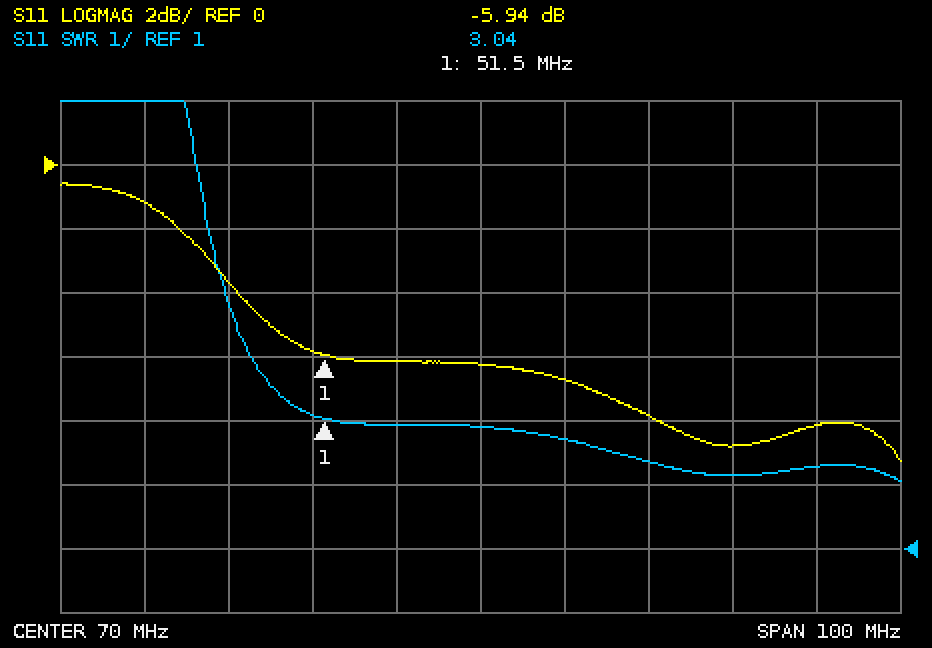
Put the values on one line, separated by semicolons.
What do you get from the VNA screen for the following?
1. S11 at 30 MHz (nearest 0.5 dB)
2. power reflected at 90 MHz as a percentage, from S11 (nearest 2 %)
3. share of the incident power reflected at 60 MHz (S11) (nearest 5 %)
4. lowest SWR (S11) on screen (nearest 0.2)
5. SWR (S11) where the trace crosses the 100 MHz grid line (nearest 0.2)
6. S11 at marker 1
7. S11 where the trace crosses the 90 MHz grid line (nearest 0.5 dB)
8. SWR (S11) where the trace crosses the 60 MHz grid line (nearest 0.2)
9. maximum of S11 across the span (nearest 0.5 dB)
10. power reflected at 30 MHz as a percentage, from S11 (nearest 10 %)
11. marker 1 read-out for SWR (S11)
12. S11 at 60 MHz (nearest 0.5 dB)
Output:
-1.0 dB; 16 %; 25 %; 2.0; 2.2; -5.94 dB; -8.0 dB; 3.0; -0.5 dB; 80 %; 3.04; -6.0 dB
